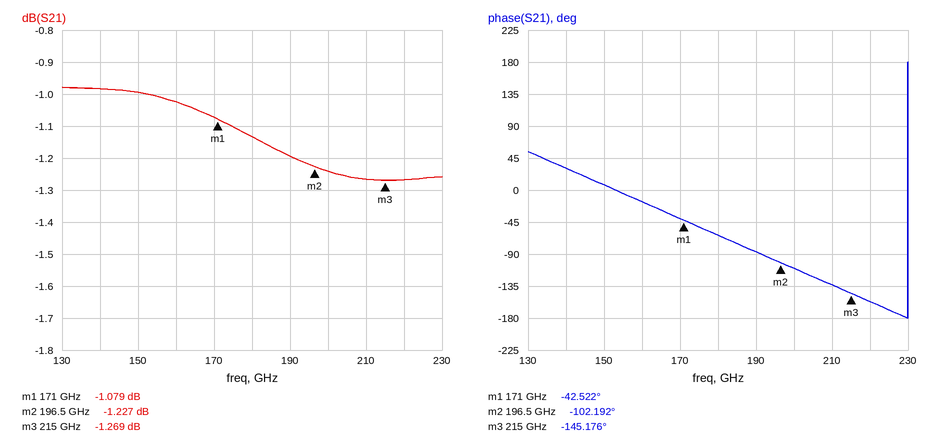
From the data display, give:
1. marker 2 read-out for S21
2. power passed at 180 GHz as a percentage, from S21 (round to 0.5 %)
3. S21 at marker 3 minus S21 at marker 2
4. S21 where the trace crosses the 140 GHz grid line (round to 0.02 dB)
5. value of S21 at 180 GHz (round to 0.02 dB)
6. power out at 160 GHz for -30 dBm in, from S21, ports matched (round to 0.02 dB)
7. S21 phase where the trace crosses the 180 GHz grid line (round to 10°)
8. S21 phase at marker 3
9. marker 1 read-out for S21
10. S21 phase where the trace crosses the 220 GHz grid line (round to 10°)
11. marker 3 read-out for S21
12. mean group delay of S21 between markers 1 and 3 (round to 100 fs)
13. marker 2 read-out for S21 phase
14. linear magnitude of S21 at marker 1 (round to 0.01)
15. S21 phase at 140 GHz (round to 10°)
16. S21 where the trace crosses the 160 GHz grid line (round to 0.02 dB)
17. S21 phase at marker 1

-1.227 dB
77.0 %
-0.042 dB
-0.98 dB
-1.14 dB
-31.02 dBm
-60°
-145.176°
-1.079 dB
-160°
-1.269 dB
6.5 ps
-102.192°
0.88
30°
-1.02 dB
-42.522°
